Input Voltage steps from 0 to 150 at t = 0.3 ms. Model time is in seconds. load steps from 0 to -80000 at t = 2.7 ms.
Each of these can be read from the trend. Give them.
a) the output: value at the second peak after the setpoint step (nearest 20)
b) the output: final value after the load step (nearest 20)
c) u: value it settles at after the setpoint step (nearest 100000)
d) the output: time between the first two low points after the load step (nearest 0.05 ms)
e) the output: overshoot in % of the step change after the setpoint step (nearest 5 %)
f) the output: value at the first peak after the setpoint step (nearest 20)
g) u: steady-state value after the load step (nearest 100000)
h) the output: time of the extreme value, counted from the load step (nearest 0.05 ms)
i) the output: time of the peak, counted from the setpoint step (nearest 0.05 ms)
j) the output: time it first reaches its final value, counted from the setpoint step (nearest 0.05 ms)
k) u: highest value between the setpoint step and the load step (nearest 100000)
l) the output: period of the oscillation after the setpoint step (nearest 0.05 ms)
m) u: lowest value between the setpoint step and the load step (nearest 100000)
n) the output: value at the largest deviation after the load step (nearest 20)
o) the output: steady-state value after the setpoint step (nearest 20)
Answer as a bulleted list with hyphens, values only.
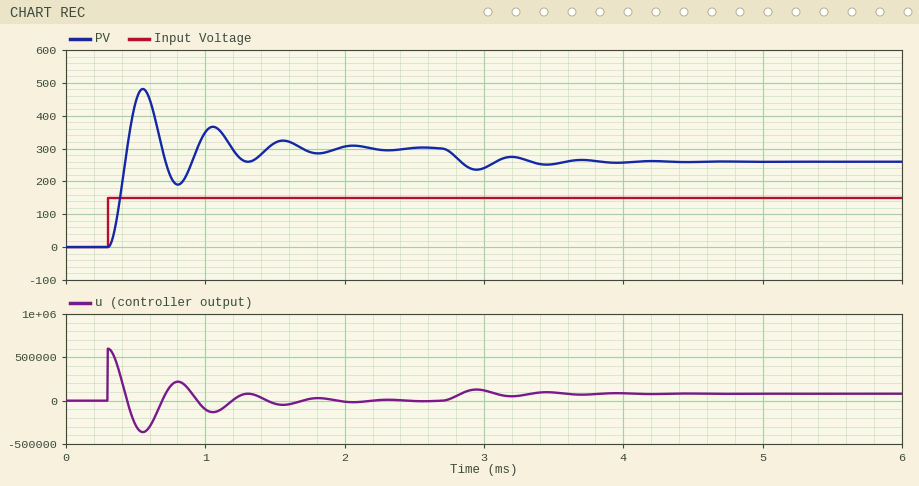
- 360
- 260
- 0
- 0.50 ms
- 60 %
- 480
- 100000
- 0.25 ms
- 0.25 ms
- 0.15 ms
- 600000
- 0.50 ms
- -400000
- 240
- 300
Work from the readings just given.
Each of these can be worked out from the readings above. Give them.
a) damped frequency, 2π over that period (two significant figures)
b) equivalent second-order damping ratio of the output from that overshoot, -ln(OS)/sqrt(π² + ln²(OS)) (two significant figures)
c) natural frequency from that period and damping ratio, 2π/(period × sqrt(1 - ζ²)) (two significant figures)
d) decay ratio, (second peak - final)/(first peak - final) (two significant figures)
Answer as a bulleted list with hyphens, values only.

- 13 rad/ms
- 0.16
- 13 rad/ms
- 0.33
